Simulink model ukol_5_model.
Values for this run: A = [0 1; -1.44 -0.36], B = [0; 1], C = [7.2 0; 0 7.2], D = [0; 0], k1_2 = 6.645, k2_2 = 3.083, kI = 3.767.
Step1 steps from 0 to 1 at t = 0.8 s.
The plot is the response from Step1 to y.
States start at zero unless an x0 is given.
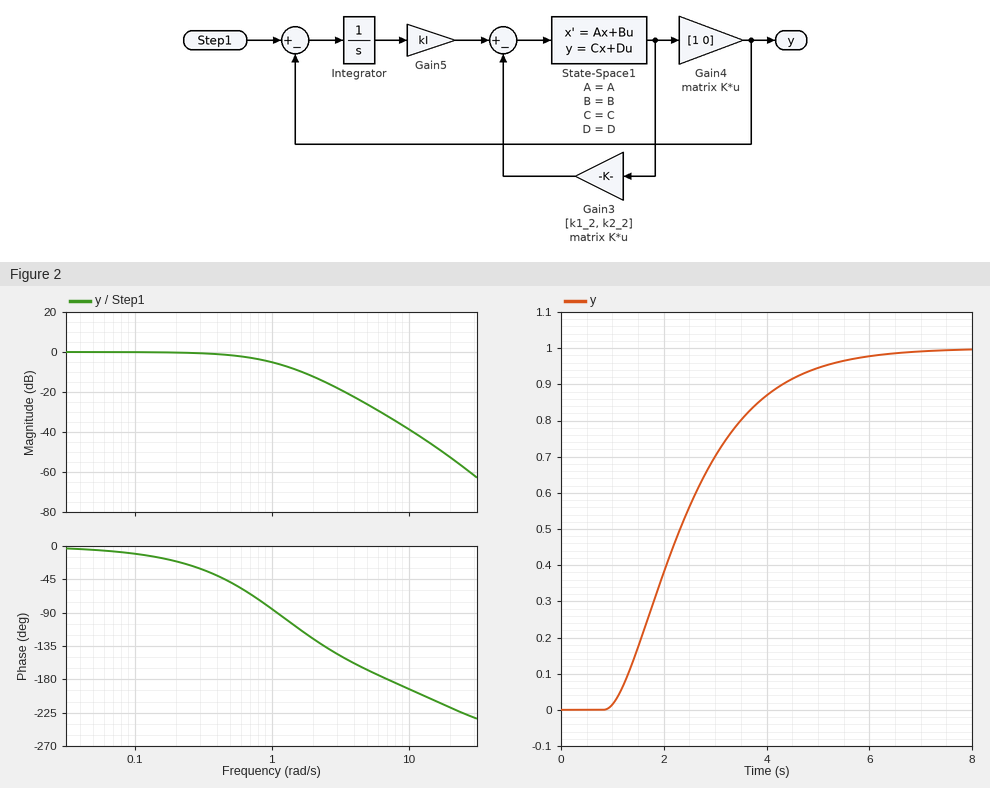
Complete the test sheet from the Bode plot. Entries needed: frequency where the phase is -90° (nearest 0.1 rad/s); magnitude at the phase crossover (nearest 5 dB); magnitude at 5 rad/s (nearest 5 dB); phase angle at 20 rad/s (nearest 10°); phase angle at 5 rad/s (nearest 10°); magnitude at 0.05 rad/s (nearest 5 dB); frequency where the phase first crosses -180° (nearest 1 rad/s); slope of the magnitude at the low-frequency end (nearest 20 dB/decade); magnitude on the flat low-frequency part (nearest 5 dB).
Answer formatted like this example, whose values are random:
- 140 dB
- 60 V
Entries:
- 1.1 rad/s
- -30 dB
- -25 dB
- -220°
- -170°
- 0 dB
- 7 rad/s
- 0 dB/decade
- 0 dB
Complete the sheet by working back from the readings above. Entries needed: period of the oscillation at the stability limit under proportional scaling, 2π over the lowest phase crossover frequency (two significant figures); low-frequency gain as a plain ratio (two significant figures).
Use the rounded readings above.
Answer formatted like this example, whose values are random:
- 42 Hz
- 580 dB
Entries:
- 0.90 s
- 1.0
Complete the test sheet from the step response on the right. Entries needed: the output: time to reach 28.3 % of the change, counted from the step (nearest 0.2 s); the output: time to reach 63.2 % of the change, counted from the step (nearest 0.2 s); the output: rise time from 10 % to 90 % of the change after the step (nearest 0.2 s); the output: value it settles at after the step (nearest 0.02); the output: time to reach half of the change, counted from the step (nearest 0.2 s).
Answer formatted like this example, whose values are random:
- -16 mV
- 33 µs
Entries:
- 1.0 s
- 2.0 s
- 3.0 s
- 1.00
- 1.6 s
